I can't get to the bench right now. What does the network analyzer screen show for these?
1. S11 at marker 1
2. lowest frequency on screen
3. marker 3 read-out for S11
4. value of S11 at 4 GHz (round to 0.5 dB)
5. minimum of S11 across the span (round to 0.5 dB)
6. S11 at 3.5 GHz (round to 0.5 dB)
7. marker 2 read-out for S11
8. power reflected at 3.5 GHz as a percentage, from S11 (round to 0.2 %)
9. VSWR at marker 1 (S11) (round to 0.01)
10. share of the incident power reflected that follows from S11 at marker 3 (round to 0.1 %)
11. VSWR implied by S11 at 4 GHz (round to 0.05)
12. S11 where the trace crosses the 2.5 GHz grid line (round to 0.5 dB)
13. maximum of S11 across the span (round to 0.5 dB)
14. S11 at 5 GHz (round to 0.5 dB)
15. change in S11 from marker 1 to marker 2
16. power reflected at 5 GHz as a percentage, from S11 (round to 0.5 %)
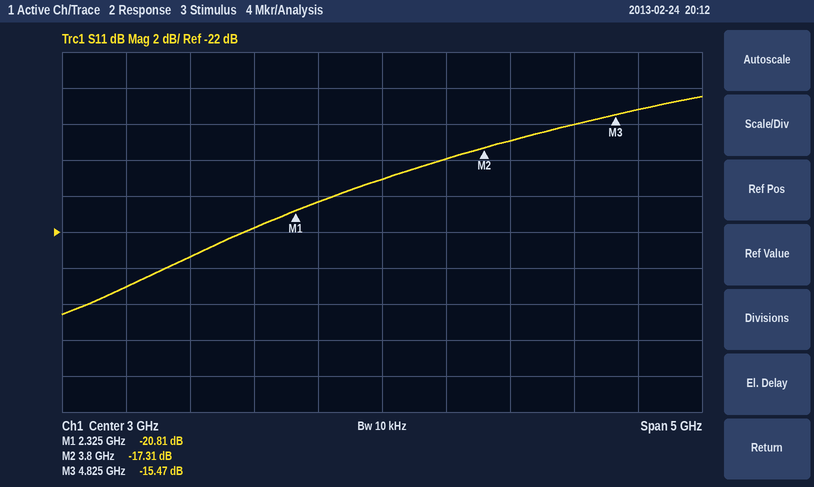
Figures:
-20.81 dB
500 MHz
-15.47 dB
-17.0 dB
-26.5 dB
-18.0 dB
-17.31 dB
1.6 %
1.20
2.8 %
1.35
-20.5 dB
-14.5 dB
-15.0 dB
3.50 dB
3.0 %
